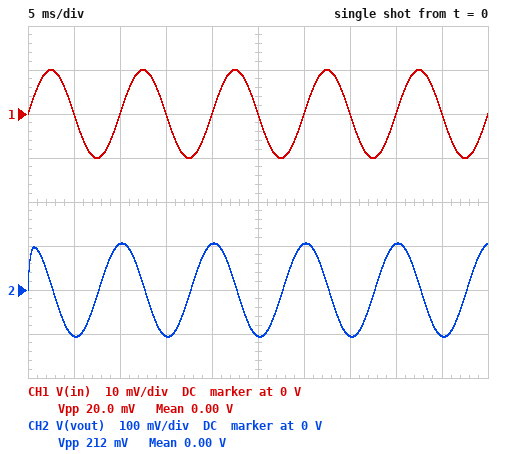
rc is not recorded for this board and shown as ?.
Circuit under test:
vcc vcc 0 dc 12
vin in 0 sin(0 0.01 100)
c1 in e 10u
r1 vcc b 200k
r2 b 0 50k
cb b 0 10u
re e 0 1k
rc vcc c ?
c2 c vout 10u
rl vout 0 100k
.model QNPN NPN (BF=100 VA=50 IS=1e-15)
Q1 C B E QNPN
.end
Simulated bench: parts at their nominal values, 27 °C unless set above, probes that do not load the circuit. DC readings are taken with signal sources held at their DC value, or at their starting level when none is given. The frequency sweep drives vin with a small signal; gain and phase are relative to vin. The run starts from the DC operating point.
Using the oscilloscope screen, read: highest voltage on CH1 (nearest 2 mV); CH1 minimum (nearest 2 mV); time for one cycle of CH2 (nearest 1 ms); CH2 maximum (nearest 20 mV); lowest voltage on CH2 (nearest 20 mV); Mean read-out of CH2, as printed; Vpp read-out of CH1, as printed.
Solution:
10 mV
-10 mV
10 ms
100 mV
-100 mV
0.00 V
20.0 mV
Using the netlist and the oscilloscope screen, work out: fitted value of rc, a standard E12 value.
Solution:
1.8 kΩ
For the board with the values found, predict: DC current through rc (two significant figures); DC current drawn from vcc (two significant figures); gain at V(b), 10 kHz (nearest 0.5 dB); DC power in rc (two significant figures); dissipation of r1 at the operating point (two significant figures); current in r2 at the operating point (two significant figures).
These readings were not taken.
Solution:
1.2 mA
1.3 mA
-63.5 dB
2.8 mW
500 µW
39 µA
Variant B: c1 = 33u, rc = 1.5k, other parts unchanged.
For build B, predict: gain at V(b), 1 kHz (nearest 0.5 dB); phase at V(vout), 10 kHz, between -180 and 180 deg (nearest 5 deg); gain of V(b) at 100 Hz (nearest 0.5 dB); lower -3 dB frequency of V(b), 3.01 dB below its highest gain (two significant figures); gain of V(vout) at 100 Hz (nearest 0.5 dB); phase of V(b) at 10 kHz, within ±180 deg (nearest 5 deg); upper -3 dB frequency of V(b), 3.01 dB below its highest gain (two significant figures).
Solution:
-44.0 dB
0 deg
-32.0 dB
520 mHz
28.5 dB
-90 deg
240 Hz
